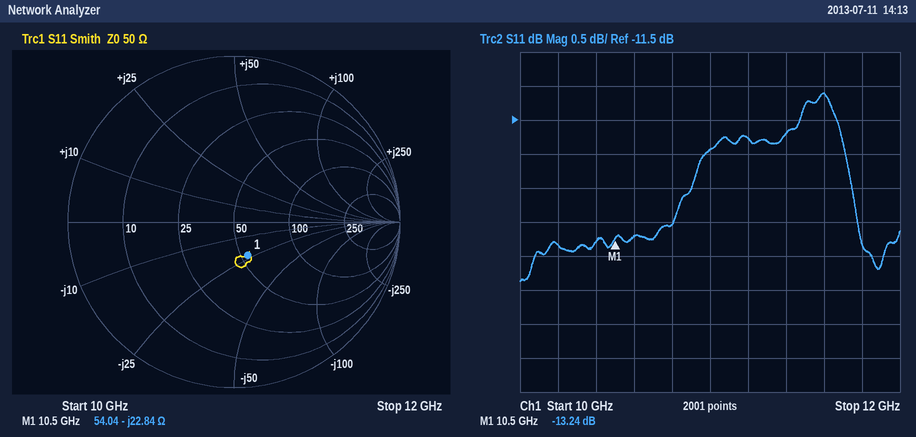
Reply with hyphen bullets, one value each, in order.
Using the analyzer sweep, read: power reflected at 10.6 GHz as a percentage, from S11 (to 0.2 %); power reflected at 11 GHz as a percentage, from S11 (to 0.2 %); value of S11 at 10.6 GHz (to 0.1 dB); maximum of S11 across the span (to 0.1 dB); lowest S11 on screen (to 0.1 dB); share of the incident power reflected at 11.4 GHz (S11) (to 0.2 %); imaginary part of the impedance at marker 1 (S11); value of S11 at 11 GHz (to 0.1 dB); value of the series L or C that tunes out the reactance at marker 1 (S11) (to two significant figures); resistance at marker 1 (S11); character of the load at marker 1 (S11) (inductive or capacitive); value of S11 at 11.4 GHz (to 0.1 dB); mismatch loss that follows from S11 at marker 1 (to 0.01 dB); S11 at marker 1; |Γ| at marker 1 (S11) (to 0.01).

- 4.8 %
- 6.4 %
- -13.2 dB
- -11.1 dB
- -13.9 dB
- 6.8 %
- -22.84 Ω
- -11.9 dB
- 350 pH
- 54.04 Ω
- capacitive
- -11.7 dB
- 0.21 dB
- -13.24 dB
- 0.22
